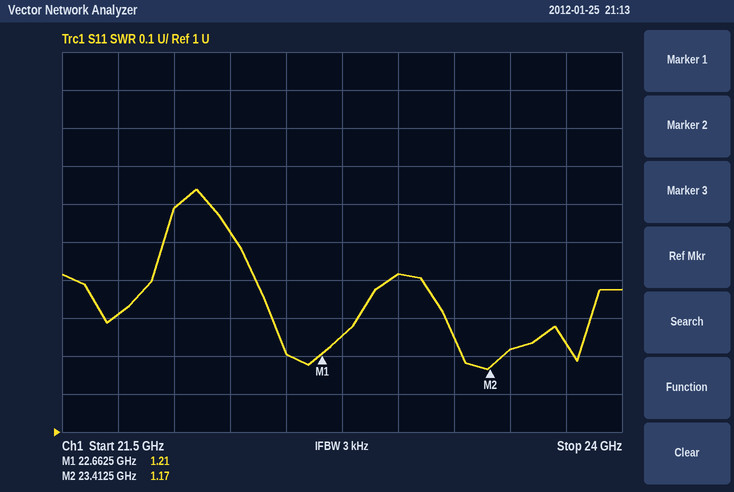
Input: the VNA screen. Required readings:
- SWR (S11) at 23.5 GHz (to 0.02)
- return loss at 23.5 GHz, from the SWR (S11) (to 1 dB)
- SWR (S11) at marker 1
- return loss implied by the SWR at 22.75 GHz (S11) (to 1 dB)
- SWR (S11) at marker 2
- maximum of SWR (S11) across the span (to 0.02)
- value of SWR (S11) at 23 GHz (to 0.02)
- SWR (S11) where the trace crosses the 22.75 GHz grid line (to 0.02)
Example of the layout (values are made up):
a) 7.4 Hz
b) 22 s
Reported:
a) 1.22
b) 20 dB
c) 1.21
d) 19 dB
e) 1.17
f) 1.64
g) 1.42
h) 1.26
